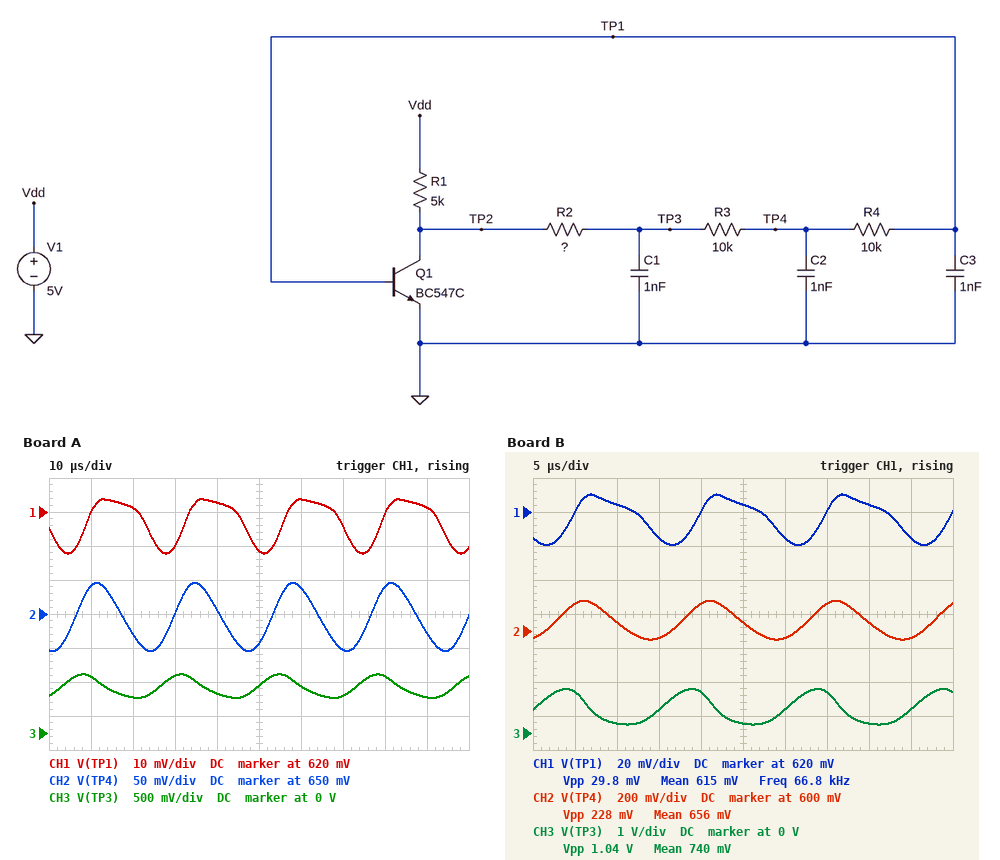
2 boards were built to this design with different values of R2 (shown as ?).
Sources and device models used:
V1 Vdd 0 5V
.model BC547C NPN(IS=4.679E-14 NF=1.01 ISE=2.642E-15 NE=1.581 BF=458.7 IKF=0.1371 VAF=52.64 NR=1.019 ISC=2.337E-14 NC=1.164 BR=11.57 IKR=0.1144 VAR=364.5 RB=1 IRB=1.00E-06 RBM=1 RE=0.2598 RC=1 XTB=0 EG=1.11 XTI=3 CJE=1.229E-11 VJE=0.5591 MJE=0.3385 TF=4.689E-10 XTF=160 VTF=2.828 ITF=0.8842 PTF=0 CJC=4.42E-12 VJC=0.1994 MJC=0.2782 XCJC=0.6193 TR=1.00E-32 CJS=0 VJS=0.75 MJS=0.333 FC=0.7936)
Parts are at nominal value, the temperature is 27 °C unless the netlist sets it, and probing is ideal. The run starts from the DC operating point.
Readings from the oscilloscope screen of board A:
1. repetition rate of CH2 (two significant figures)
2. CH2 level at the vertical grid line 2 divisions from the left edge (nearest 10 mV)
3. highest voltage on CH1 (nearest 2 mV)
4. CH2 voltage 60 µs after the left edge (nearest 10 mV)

43 kHz
620 mV
624 mV
690 mV
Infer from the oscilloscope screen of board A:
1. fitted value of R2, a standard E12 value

15 kΩ
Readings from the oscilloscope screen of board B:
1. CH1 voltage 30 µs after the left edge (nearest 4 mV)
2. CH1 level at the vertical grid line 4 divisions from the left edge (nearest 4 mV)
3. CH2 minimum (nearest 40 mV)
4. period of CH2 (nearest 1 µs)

604 mV
620 mV
560 mV
15 µs
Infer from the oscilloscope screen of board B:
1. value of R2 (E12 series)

2.2 kΩ
